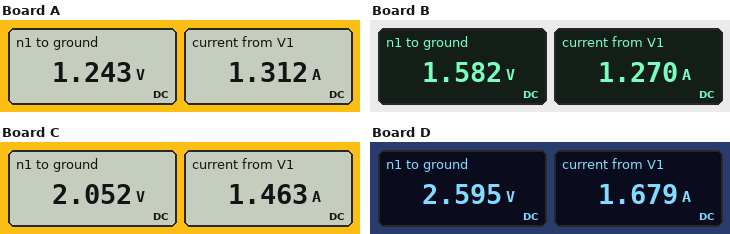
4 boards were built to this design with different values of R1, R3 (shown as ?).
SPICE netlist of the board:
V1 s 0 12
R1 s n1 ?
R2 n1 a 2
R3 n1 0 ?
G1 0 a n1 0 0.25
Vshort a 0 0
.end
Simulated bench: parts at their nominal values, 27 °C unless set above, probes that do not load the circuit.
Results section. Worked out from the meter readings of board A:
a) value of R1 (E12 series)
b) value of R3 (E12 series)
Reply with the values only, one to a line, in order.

8.2 Ω
1.8 Ω
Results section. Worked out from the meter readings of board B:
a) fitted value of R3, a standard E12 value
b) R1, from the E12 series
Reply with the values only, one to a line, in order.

3.3 Ω
8.2 Ω
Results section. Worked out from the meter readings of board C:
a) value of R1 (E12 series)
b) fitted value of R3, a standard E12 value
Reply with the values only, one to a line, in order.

6.8 Ω
4.7 Ω
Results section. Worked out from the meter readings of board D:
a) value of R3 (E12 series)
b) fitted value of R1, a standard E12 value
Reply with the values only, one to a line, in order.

6.8 Ω
5.6 Ω
